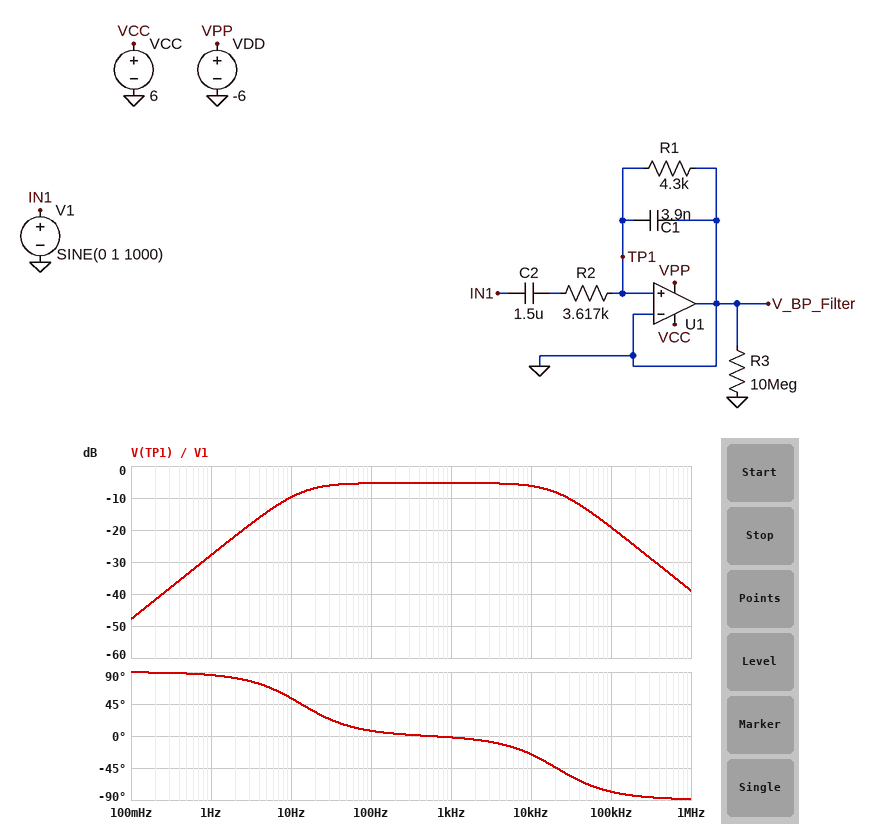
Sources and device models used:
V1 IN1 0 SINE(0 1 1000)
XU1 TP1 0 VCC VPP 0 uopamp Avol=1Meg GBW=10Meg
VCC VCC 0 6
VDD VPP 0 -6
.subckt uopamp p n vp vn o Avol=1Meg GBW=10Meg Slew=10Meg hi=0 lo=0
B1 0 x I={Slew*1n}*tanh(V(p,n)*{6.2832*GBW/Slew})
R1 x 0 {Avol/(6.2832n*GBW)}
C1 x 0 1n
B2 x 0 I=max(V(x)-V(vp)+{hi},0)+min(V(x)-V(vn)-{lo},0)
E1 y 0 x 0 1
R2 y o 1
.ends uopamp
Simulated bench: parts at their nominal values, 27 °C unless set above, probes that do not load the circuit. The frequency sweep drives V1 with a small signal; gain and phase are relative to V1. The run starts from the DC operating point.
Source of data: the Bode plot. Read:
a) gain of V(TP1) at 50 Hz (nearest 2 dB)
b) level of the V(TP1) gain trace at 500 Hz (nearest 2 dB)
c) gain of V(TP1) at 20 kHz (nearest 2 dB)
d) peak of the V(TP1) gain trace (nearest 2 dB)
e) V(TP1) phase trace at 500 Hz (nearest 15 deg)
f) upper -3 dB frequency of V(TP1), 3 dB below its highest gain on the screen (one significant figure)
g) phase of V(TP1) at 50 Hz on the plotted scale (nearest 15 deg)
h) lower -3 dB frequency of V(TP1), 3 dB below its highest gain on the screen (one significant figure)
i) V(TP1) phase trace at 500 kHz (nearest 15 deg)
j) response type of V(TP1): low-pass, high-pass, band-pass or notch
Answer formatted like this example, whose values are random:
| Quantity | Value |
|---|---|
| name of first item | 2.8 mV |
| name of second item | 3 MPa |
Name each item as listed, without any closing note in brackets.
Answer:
| Quantity | Value |
|---|---|
| gain of V(TP1) at 50 Hz | -6 dB |
| level of the V(TP1) gain trace at 500 Hz | -6 dB |
| gain of V(TP1) at 20 kHz | -8 dB |
| peak of the V(TP1) gain trace | -6 dB |
| V(TP1) phase trace at 500 Hz | 0 deg |
| upper -3 dB frequency of V(TP1), 3 dB below its highest gain on the screen | 20 kHz |
| phase of V(TP1) at 50 Hz on the plotted scale | 15 deg |
| lower -3 dB frequency of V(TP1), 3 dB below its highest gain on the screen | 10 Hz |
| V(TP1) phase trace at 500 kHz | -90 deg |
| response type of V(TP1): low-pass, high-pass, band-pass or notch | band-pass |
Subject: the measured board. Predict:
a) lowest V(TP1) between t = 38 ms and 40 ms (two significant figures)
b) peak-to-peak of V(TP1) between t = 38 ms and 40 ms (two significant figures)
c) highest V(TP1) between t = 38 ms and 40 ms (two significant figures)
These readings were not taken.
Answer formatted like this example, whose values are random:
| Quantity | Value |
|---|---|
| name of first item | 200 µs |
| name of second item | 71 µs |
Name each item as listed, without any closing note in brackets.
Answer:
| Quantity | Value |
|---|---|
| lowest V(TP1) between t = 38 ms and 40 ms | -540 mV |
| peak-to-peak of V(TP1) between t = 38 ms and 40 ms | 1.1 V |
| highest V(TP1) between t = 38 ms and 40 ms | 540 mV |
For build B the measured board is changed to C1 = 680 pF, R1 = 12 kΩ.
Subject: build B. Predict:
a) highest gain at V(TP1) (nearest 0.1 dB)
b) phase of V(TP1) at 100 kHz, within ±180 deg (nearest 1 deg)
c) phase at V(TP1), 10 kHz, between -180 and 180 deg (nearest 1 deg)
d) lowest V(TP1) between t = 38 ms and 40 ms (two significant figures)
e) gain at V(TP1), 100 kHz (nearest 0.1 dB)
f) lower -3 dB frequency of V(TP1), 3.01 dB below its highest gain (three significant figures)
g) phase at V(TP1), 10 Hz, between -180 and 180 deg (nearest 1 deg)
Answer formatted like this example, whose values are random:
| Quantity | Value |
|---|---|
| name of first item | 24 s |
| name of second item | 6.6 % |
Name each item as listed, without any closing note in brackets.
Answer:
| Quantity | Value |
|---|---|
| highest gain at V(TP1) | -2.3 dB |
| phase of V(TP1) at 100 kHz, within ±180 deg | -50 deg |
| phase at V(TP1), 10 kHz, between -180 and 180 deg | -7 deg |
| lowest V(TP1) between t = 38 ms and 40 ms | -770 mV |
| gain at V(TP1), 100 kHz | -6.1 dB |
| lower -3 dB frequency of V(TP1), 3.01 dB below its highest gain | 6.79 Hz |
| phase at V(TP1), 10 Hz, between -180 and 180 deg | 34 deg |
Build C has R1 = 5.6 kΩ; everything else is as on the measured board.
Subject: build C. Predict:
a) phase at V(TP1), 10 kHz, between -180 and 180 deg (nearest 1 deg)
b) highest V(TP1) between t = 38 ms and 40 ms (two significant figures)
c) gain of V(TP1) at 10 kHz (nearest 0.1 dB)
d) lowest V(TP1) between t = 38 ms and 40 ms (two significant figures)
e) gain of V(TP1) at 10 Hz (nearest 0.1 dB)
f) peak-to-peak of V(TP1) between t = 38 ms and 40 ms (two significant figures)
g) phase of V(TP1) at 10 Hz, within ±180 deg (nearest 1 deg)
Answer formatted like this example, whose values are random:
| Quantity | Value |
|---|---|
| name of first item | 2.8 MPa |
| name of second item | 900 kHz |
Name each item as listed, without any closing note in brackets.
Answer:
| Quantity | Value |
|---|---|
| phase at V(TP1), 10 kHz, between -180 and 180 deg | -28 deg |
| highest V(TP1) between t = 38 ms and 40 ms | 610 mV |
| gain of V(TP1) at 10 kHz | -5.4 dB |
| lowest V(TP1) between t = 38 ms and 40 ms | -610 mV |
| gain of V(TP1) at 10 Hz | -8.0 dB |
| peak-to-peak of V(TP1) between t = 38 ms and 40 ms | 1.2 V |
| phase of V(TP1) at 10 Hz, within ±180 deg | 49 deg |
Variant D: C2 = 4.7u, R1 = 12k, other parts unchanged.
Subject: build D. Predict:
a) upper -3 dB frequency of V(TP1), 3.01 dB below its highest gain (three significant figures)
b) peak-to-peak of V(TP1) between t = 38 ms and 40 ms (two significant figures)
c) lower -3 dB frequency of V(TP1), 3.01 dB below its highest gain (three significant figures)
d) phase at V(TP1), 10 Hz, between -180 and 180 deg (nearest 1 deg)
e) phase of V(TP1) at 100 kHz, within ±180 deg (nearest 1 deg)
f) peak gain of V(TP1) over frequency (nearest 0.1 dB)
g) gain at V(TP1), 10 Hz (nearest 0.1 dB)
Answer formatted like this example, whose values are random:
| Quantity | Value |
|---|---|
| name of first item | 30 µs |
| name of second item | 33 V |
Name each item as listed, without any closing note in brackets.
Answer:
| Quantity | Value |
|---|---|
| upper -3 dB frequency of V(TP1), 3.01 dB below its highest gain | 14.7 kHz |
| peak-to-peak of V(TP1) between t = 38 ms and 40 ms | 1.5 V |
| lower -3 dB frequency of V(TP1), 3.01 dB below its highest gain | 2.17 Hz |
| phase at V(TP1), 10 Hz, between -180 and 180 deg | 12 deg |
| phase of V(TP1) at 100 kHz, within ±180 deg | -82 deg |
| peak gain of V(TP1) over frequency | -2.3 dB |
| gain at V(TP1), 10 Hz | -2.5 dB |
